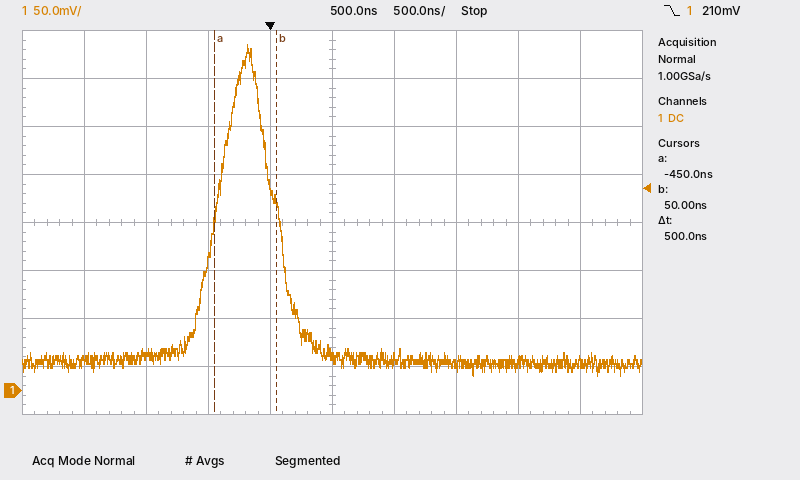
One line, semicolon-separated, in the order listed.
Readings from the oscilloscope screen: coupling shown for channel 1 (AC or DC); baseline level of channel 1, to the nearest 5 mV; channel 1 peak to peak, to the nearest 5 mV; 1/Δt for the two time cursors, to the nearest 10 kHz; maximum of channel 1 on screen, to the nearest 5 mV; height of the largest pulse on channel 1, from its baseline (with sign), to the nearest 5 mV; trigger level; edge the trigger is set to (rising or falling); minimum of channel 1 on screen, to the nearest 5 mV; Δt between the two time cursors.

DC; 30 mV; 345 mV; 2.00 MHz; 360 mV; +330 mV; 210 mV; falling; 15 mV; 500 ns
